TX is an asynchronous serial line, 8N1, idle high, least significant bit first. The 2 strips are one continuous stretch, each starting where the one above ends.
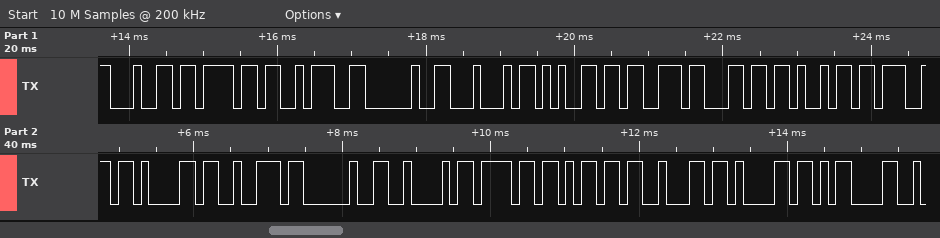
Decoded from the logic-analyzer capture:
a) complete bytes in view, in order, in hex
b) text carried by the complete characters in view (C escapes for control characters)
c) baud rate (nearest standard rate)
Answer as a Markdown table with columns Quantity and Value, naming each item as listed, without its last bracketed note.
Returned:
| Quantity | Value |
|---|---|
| complete bytes in view, in order, in hex | 64 6F 3A 20 44 65 73 6C 69 67 61 72 20 42 6F 6D 62 61 0D |
| text carried by the complete characters in view | "do: Desligar Bomba\r" |
| baud rate | 9600 baud |
